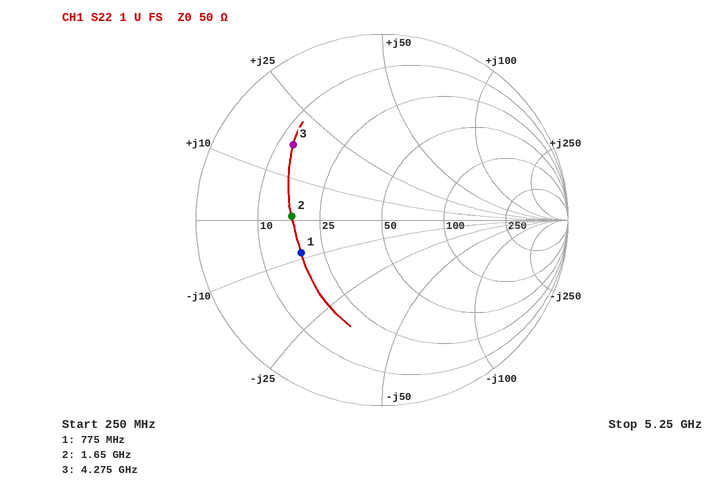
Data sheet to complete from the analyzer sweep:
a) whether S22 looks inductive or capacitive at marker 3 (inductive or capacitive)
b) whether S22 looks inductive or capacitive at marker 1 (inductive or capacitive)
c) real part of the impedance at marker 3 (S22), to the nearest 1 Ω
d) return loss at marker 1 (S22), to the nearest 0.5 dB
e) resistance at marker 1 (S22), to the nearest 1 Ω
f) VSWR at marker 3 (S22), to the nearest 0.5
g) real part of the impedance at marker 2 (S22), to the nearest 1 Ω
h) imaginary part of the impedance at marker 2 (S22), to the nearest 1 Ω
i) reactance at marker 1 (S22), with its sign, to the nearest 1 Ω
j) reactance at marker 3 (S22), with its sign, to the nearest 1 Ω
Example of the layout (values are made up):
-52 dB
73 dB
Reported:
inductive
capacitive
13 Ω
6.5 dB
19 Ω
4.5
17 Ω
+1 Ω
-8 Ω
+17 Ω
